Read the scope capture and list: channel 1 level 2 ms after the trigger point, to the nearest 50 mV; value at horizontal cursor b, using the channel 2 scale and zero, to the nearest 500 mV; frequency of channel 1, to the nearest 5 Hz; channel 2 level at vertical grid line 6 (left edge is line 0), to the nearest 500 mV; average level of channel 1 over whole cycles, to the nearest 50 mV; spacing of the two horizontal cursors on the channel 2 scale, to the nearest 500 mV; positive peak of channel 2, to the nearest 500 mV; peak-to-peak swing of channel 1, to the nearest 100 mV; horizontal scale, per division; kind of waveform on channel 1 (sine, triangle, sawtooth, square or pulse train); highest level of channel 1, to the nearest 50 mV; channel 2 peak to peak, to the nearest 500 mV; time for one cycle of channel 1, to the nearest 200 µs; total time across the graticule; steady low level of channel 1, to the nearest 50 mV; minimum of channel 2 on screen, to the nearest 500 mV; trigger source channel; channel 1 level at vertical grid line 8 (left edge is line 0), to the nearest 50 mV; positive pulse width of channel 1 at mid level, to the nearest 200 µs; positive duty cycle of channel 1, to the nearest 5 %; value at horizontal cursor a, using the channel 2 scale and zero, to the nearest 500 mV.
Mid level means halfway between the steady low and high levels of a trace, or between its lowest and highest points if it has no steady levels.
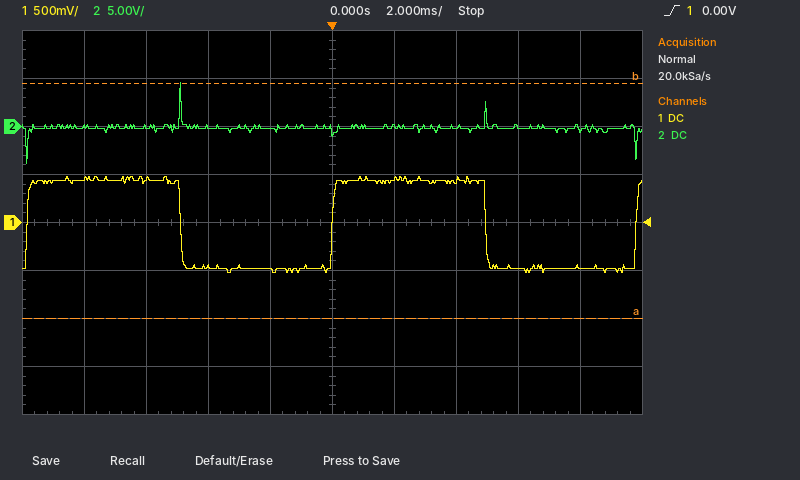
450 mV
4.5 V
100 Hz
0.0 V
0 mV
24.5 V
4.5 V
1.00 V
2 ms
square
500 mV
8.5 V
9.8 ms
20 ms
-500 mV
-4.0 V
channel 1
-500 mV
5.0 ms
50 %
-20.0 V
